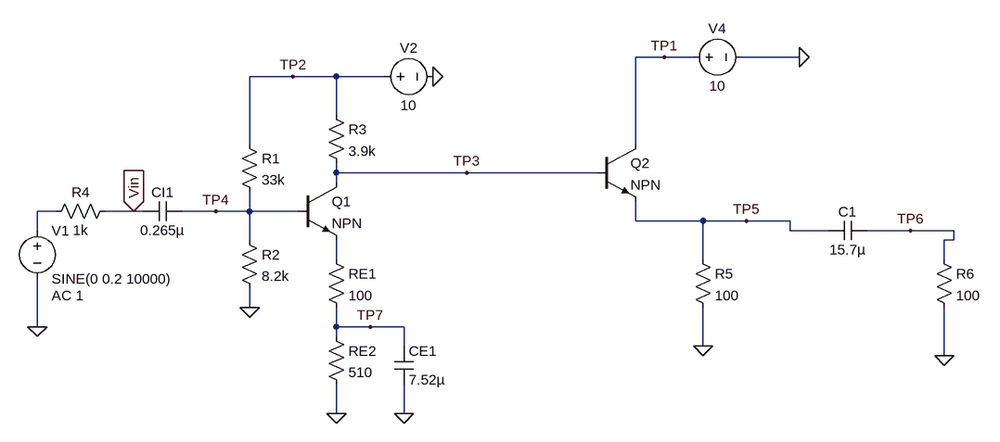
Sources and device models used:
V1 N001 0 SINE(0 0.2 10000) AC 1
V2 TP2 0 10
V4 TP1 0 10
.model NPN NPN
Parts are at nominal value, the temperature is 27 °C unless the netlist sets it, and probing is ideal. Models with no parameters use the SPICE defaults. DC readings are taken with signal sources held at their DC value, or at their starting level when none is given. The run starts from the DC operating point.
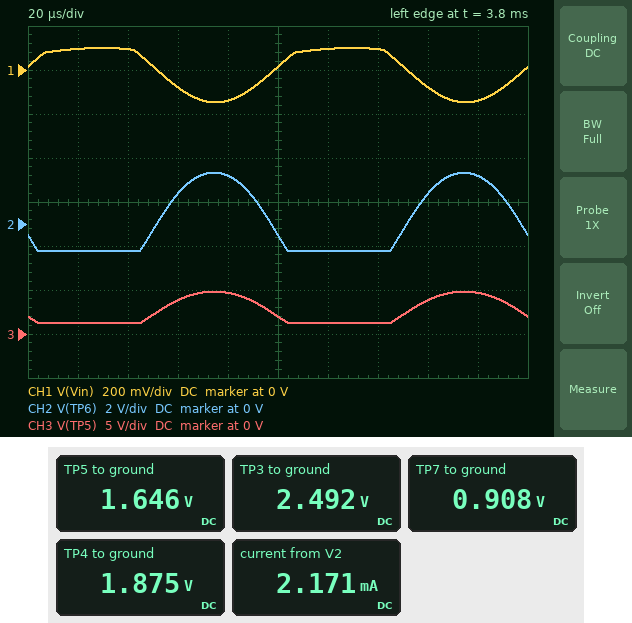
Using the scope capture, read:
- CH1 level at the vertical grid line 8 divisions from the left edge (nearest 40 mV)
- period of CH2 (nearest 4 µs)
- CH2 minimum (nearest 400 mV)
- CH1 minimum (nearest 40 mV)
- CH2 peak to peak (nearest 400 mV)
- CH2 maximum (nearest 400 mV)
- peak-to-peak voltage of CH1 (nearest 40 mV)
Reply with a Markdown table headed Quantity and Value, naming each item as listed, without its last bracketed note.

| Quantity | Value |
|---|---|
| CH1 level at the vertical grid line 8 divisions from the left edge | -80 mV |
| period of CH2 | 100 µs |
| CH2 minimum | -1.2 V |
| CH1 minimum | -160 mV |
| CH2 peak to peak | 3.6 V |
| CH2 maximum | 2.4 V |
| peak-to-peak voltage of CH1 | 240 mV |
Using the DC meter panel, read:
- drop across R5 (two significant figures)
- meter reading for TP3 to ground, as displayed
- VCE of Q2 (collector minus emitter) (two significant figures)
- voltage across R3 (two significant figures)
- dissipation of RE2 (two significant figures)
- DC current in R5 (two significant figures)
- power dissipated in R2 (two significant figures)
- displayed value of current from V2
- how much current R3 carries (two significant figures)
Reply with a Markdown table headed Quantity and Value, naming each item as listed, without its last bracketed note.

| Quantity | Value |
|---|---|
| drop across R5 | 1.6 V |
| meter reading for TP3 to ground, as displayed | 2.492 V |
| VCE of Q2 (collector minus emitter) | 8.4 V |
| voltage across R3 | 7.5 V |
| dissipation of RE2 | 1.6 mW |
| DC current in R5 | 16 mA |
| power dissipated in R2 | 430 µW |
| displayed value of current from V2 | 2.171 mA |
| how much current R3 carries | 1.9 mA |
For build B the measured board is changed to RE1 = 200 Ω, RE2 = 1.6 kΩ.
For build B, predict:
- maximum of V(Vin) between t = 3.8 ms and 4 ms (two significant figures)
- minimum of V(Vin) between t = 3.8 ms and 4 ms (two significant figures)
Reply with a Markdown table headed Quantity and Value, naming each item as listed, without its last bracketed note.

| Quantity | Value |
|---|---|
| maximum of V(Vin) between t = 3.8 ms and 4 ms | 170 mV |
| minimum of V(Vin) between t = 3.8 ms and 4 ms | -170 mV |
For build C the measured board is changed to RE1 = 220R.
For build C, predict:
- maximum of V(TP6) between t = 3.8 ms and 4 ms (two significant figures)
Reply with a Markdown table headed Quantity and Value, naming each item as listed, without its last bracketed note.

| Quantity | Value |
|---|---|
| maximum of V(TP6) between t = 3.8 ms and 4 ms | 1.5 V |
